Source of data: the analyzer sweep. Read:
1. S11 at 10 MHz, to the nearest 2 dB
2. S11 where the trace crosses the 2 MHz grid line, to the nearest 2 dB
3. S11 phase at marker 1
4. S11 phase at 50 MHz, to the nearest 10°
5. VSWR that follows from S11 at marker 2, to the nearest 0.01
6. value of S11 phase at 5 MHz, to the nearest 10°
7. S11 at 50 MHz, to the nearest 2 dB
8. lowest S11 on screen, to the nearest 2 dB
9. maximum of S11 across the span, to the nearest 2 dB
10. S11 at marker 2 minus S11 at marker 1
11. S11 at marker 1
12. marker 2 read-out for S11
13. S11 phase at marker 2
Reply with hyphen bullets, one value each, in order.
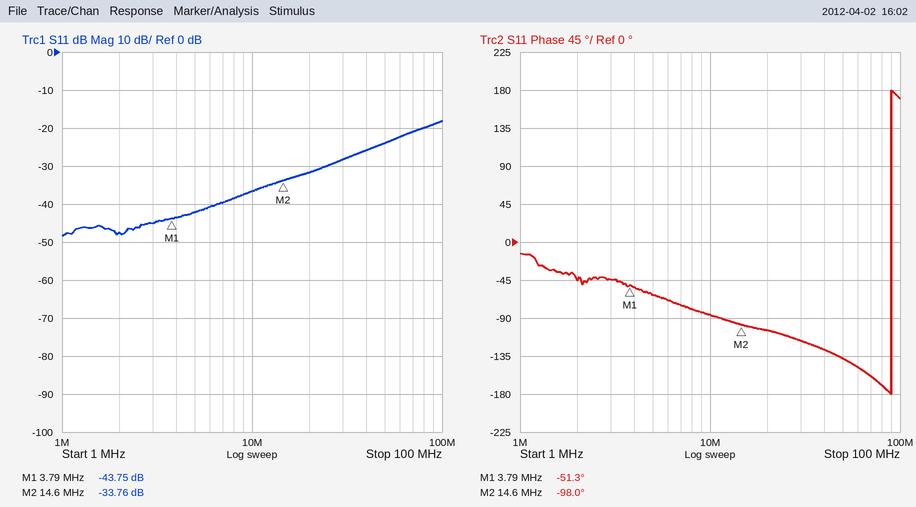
- -36 dB
- -48 dB
- -51.3°
- -140°
- 1.04
- -60°
- -24 dB
- -48 dB
- -18 dB
- 9.99 dB
- -43.75 dB
- -33.76 dB
- -98.0°
